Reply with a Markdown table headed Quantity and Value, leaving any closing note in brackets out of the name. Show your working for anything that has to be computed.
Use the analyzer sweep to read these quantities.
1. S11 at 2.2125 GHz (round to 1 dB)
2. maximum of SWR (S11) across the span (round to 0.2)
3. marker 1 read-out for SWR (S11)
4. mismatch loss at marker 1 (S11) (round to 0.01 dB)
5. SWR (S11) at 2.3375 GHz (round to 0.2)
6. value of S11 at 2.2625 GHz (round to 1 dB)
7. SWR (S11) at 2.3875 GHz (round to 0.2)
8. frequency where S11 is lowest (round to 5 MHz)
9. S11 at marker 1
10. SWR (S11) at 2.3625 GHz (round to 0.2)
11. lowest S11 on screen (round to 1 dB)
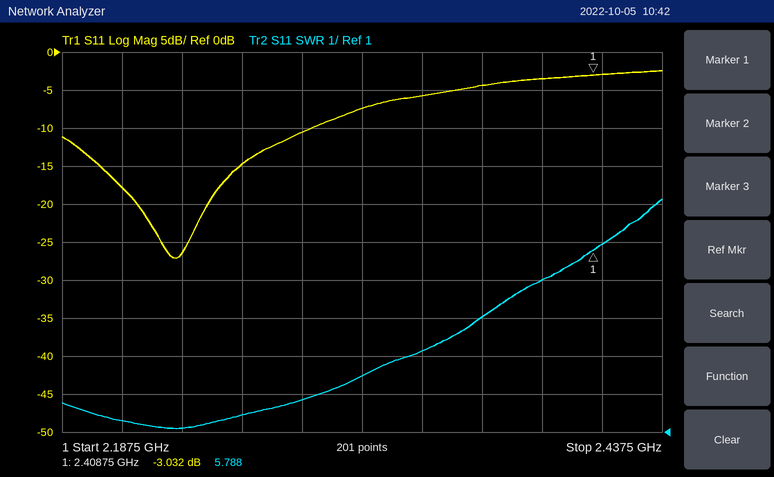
| Quantity | Value |
|---|---|
| S11 at 2.2125 GHz | -18 dB |
| maximum of SWR (S11) across the span | 7.2 |
| marker 1 read-out for SWR | 5.788 |
| mismatch loss at marker 1 (S11) | −10 log10(1 − 10^(-3.032/10)) ≈ 2.99 dB |
| SWR (S11) at 2.3375 GHz | 3.2 |
| value of S11 at 2.2625 GHz | -15 dB |
| SWR (S11) at 2.3875 GHz | 5.0 |
| frequency where S11 is lowest | 2.235 GHz |
| S11 at marker 1 | -3.032 dB |
| SWR (S11) at 2.3625 GHz | 4.0 |
| lowest S11 on screen | -27 dB |
